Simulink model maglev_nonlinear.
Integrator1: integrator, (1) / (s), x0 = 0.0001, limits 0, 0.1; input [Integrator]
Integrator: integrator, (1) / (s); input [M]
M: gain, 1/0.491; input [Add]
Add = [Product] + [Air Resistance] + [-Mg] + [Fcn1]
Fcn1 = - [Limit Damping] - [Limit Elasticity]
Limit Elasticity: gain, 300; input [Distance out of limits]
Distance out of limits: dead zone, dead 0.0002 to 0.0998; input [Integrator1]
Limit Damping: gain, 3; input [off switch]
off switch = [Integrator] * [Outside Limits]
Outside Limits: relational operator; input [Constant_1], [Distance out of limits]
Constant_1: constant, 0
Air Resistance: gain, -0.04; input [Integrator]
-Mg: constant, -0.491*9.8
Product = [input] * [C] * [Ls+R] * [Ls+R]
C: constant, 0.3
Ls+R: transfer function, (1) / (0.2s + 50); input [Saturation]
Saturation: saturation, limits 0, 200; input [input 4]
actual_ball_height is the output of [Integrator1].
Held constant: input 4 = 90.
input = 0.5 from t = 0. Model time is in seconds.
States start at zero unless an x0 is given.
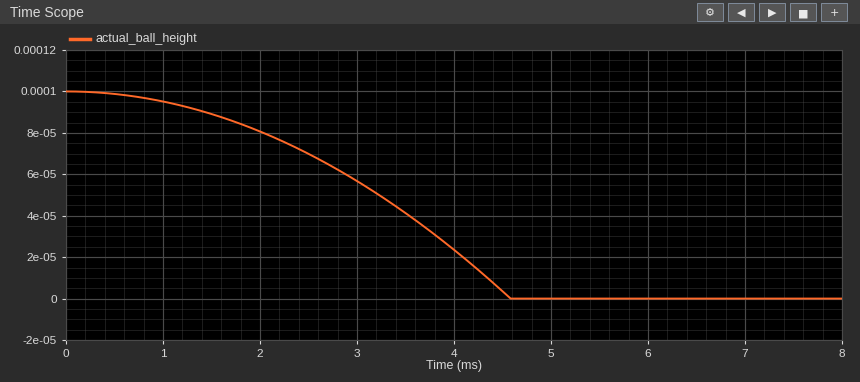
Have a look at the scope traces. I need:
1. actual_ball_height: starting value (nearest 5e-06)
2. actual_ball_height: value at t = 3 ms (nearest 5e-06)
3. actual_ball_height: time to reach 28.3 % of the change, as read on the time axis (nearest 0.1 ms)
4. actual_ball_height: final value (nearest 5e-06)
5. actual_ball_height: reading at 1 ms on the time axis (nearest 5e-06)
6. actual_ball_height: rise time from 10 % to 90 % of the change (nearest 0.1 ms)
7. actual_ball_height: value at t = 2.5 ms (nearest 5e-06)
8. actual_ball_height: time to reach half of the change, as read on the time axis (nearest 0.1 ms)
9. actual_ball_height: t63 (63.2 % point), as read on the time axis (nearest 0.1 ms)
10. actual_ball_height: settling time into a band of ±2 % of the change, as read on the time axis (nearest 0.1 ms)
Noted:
0.000100
0.000055
2.4 ms
0.000000
0.000095
2.9 ms
0.000070
3.2 ms
3.6 ms
4.5 ms
